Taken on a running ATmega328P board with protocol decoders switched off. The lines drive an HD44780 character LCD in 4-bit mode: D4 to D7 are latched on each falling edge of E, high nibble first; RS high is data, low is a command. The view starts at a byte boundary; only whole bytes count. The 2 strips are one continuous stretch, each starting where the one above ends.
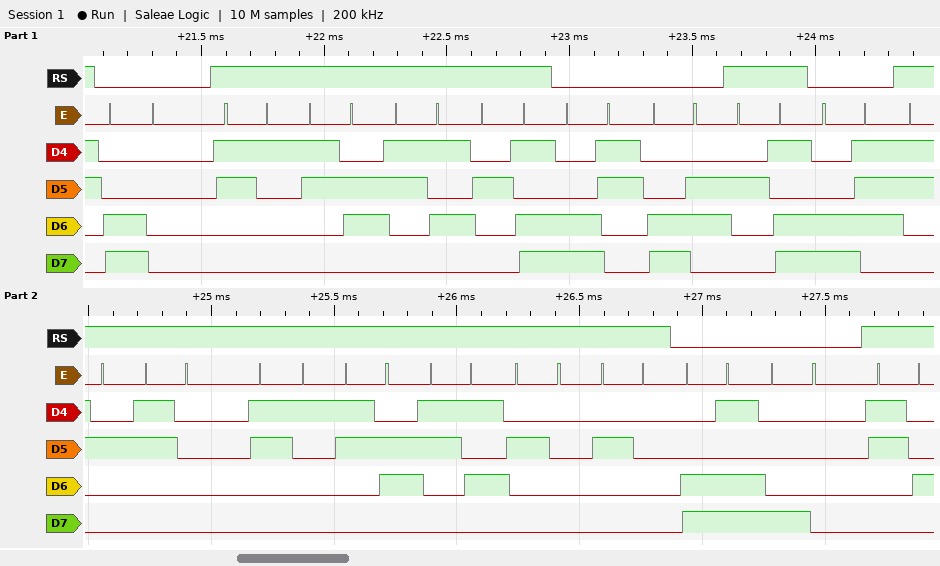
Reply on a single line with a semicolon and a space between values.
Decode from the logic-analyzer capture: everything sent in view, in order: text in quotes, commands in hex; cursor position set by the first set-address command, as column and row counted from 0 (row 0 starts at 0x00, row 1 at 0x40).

0xC0 "165-" 0xC3 0xC6 "-" 0xC7 "20165  " 0xCD 0x80 "4"; column 0, row 1
